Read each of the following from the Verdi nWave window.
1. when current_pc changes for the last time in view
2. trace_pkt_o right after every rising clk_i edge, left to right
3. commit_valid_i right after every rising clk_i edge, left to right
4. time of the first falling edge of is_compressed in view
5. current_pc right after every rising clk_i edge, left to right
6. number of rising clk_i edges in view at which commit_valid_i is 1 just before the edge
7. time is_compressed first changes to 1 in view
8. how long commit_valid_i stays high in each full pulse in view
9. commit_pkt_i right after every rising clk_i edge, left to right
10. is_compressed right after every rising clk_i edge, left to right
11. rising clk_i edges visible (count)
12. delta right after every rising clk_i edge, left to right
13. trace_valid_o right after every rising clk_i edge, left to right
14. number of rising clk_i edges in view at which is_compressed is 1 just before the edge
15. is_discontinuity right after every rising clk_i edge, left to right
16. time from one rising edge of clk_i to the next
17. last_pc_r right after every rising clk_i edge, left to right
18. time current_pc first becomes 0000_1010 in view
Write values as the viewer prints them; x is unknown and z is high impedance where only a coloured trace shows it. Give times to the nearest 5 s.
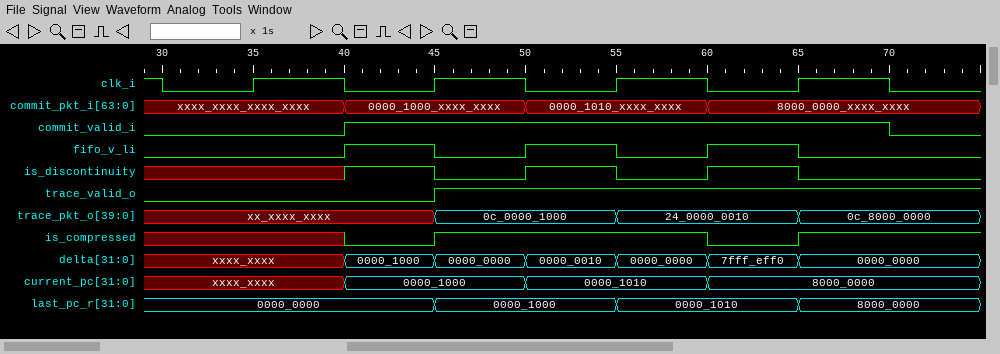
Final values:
60 s
xx_xxxx_xxxx, 0c_0000_1000, 24_0000_0010, 0c_8000_0000
0 1 1 1
60 s
xxxx_xxxx, 0000_1000, 0000_1010, 8000_0000
3
45 s
30 s
xxxx_xxxx_xxxx_xxxx, 0000_1000_xxxx_xxxx, 0000_1010_xxxx_xxxx, 8000_0000_xxxx_xxxx
x 1 1 1
4
xxxx_xxxx, 0000_0000, 0000_0000, 0000_0000
0 1 1 1
1
x 0 0 0
10 s
0000_0000, 0000_1000, 0000_1010, 8000_0000
50 s
